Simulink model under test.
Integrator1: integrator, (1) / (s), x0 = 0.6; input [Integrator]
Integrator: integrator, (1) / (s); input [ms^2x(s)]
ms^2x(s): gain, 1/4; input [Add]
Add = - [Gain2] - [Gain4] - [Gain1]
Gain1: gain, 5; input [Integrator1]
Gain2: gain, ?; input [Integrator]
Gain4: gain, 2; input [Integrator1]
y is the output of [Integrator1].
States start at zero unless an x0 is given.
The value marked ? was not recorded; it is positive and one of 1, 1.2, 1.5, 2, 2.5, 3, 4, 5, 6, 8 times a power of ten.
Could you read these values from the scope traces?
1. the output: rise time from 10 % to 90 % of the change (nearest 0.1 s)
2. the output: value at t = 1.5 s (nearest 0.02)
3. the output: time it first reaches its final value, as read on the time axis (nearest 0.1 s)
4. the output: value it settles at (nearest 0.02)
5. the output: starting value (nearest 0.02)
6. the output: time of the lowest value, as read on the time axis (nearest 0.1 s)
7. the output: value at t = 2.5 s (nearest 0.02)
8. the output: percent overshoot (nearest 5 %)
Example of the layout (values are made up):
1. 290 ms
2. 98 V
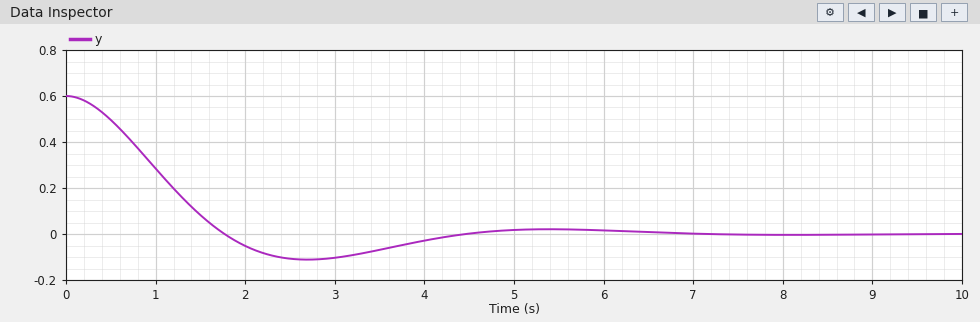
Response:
1. 1.2 s
2. 0.08
3. 1.8 s
4. 0.00
5. 0.60
6. 2.7 s
7. -0.10
8. 20 %
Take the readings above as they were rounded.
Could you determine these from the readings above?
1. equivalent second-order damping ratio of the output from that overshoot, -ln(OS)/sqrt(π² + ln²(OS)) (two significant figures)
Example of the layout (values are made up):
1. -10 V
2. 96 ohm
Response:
1. 0.46
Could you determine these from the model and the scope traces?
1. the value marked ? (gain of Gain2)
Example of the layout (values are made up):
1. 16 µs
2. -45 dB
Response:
1. 5
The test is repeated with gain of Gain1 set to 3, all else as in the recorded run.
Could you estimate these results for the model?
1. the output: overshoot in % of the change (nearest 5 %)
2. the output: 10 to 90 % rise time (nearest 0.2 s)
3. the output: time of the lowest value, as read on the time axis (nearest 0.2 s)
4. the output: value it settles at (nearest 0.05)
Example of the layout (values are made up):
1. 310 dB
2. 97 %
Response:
1. 10 %
2. 1.6 s
3. 3.4 s
4. 0.00
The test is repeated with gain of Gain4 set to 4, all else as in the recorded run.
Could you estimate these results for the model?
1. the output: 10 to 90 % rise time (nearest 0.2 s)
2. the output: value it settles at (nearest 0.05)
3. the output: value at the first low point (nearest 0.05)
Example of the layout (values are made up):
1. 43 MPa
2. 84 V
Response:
1. 1.0 s
2. 0.00
3. -0.15
